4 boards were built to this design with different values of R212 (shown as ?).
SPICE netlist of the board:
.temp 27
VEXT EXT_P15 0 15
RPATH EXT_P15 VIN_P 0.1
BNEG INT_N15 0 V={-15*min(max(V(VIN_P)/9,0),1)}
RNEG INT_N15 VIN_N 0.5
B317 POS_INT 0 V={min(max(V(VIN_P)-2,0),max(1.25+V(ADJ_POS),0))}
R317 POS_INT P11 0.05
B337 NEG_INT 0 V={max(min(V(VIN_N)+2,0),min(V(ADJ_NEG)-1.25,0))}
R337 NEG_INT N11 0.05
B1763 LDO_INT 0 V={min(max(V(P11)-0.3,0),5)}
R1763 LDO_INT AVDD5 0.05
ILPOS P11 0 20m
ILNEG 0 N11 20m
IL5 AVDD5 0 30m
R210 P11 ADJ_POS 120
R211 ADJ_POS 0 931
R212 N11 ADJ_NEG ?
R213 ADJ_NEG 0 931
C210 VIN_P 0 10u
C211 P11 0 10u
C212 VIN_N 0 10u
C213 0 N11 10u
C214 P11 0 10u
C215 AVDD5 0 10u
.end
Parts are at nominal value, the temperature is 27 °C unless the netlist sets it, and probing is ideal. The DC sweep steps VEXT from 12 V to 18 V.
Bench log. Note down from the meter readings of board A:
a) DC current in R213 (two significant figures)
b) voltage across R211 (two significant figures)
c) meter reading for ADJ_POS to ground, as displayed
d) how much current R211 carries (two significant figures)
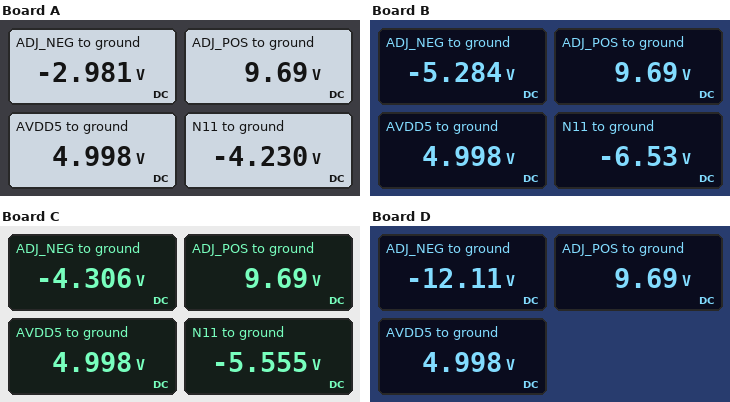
3.2 mA
9.7 V
9.69 V
10 mA
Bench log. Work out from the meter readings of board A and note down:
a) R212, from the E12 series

390 Ω
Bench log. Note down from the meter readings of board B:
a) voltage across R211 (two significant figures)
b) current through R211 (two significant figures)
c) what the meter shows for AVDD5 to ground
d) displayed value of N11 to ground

9.7 V
10 mA
4.998 V
-6.53 V
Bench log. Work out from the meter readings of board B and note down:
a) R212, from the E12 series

220 Ω
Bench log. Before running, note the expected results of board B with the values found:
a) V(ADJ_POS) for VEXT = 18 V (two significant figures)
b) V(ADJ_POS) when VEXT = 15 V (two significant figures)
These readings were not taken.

9.7 V
9.7 V
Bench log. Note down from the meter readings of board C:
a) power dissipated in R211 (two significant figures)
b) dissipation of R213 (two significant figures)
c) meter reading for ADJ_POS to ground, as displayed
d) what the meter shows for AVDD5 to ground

100 mW
20 mW
9.69 V
4.998 V
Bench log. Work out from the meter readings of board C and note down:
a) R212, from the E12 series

270 Ω
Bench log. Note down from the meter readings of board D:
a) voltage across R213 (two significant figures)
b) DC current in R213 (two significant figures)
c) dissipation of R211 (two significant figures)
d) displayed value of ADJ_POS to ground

12 V
13 mA
100 mW
9.69 V
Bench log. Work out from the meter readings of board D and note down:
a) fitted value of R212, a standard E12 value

68 Ω
